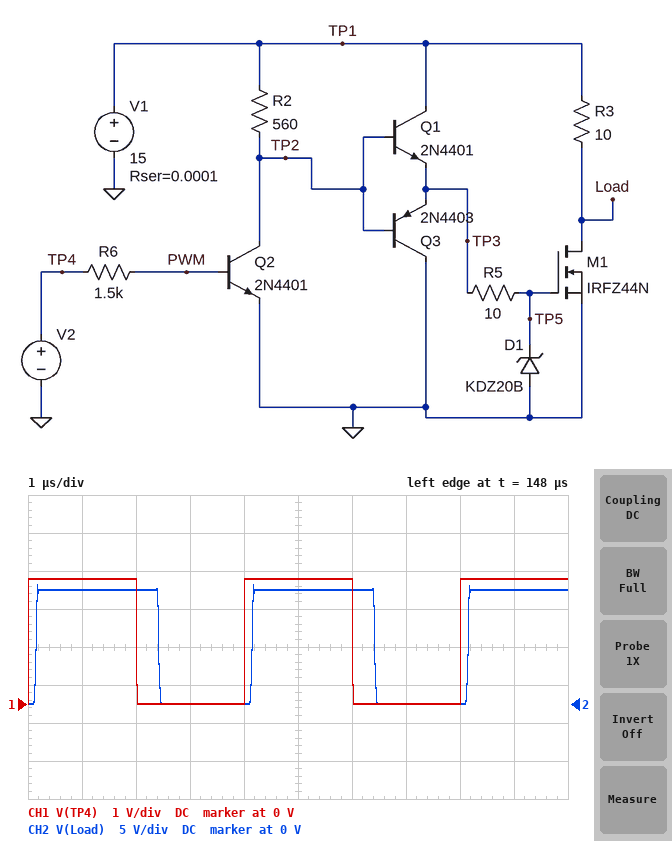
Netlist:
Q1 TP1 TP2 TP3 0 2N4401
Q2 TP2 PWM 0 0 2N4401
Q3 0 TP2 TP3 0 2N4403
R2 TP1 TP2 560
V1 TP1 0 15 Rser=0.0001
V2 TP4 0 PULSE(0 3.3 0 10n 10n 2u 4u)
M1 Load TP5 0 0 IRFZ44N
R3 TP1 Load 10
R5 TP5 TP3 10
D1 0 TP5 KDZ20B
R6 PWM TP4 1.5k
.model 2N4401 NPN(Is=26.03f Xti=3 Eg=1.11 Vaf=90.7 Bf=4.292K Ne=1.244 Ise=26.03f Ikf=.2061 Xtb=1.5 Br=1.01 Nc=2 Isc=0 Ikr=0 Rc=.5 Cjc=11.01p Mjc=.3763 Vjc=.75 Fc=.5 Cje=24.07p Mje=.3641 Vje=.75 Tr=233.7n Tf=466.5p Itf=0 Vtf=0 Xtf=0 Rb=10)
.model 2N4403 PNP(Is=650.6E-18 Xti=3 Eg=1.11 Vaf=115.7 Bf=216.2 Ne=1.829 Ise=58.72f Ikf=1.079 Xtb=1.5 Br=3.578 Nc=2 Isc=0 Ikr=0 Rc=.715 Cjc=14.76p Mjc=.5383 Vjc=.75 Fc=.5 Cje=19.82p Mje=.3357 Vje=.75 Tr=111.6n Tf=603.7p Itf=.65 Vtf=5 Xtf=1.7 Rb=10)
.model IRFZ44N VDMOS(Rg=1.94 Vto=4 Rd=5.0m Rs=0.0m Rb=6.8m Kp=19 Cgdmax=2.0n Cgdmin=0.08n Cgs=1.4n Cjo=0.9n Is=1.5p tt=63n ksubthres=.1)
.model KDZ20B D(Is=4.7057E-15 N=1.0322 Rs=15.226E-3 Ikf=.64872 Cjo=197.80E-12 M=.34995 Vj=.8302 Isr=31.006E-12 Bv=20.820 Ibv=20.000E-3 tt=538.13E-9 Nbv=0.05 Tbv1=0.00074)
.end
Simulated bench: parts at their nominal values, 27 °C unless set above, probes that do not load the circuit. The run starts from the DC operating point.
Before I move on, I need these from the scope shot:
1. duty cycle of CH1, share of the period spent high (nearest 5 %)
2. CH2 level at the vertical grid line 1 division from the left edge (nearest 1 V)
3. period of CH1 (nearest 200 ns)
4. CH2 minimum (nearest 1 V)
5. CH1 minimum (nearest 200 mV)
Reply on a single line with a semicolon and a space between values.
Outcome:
50 %; 15 V; 4.0 µs; 0 V; 0 V
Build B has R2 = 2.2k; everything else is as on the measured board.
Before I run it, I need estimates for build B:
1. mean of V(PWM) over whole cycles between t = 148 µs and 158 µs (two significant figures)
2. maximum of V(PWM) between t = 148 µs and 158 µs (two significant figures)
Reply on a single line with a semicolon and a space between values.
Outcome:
450 mV; 730 mV
